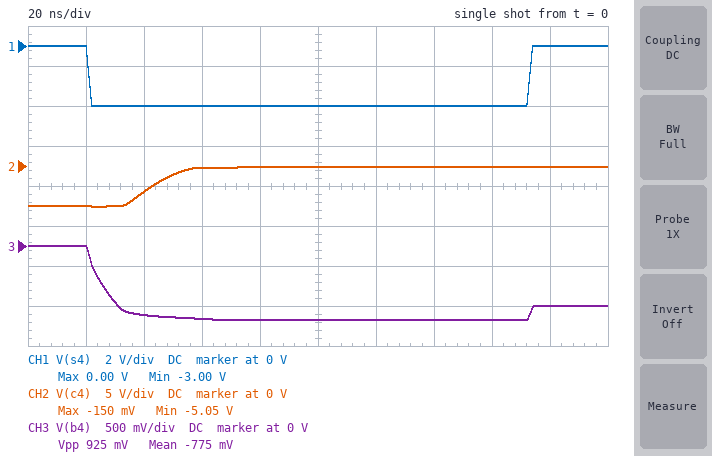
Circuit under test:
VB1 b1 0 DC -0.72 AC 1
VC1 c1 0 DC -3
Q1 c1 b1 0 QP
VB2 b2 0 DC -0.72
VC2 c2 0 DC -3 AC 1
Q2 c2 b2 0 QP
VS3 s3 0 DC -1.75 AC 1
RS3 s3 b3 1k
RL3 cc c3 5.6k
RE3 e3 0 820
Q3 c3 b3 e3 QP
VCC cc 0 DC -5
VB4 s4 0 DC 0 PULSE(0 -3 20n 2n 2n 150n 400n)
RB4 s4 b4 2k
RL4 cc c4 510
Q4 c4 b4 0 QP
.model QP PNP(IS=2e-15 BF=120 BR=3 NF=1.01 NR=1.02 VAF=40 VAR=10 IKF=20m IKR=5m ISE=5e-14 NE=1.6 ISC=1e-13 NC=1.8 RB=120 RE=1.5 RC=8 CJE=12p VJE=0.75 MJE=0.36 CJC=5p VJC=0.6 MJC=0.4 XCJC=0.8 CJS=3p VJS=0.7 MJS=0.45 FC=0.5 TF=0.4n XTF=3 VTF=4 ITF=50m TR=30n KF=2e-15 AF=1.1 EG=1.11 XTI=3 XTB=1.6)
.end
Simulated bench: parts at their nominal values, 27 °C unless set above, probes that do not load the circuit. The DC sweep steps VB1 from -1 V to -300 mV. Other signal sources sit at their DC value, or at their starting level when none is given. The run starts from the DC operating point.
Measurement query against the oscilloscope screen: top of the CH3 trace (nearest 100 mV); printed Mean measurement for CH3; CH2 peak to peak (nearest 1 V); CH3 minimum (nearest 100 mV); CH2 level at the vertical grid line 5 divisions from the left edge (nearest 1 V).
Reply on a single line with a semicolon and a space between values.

0 V; -775 mV; 5 V; -900 mV; 0 V
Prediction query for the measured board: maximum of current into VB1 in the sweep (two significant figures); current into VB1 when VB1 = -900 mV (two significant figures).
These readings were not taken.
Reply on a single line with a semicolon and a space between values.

960 µA; 470 µA
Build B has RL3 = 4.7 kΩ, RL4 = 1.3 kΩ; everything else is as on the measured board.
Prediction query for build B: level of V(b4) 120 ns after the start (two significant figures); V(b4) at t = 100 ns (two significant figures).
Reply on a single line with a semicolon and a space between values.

-900 mV; -890 mV
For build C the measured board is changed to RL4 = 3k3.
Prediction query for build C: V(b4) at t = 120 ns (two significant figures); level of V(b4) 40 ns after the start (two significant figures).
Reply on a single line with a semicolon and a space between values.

-880 mV; -830 mV
